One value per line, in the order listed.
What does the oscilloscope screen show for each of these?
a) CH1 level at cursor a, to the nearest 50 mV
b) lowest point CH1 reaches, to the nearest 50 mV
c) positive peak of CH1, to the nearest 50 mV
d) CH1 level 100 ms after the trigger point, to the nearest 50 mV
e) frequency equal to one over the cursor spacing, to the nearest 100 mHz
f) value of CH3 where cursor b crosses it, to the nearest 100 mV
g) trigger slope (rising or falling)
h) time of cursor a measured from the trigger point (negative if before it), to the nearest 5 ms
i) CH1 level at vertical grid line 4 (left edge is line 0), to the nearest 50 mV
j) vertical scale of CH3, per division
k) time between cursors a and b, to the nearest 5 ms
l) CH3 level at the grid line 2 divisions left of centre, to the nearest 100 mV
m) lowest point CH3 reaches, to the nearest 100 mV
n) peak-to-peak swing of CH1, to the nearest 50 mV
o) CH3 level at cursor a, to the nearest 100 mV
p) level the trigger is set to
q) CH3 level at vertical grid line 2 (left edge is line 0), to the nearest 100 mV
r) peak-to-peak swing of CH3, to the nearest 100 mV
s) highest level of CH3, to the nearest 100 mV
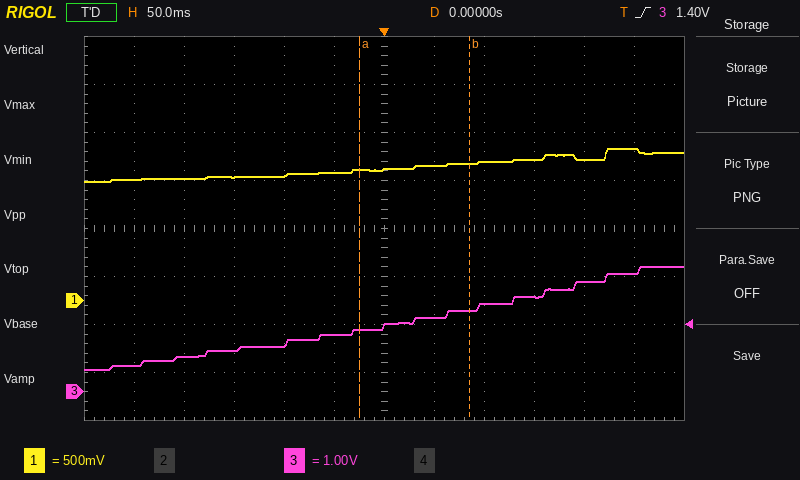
1.35 V
1.25 V
1.60 V
1.45 V
9.1 Hz
1.7 V
rising
-25 ms
1.30 V
1 V
110 ms
1.0 V
500 mV
350 mV
1.3 V
1.40 V
700 mV
2.1 V
2.6 V
